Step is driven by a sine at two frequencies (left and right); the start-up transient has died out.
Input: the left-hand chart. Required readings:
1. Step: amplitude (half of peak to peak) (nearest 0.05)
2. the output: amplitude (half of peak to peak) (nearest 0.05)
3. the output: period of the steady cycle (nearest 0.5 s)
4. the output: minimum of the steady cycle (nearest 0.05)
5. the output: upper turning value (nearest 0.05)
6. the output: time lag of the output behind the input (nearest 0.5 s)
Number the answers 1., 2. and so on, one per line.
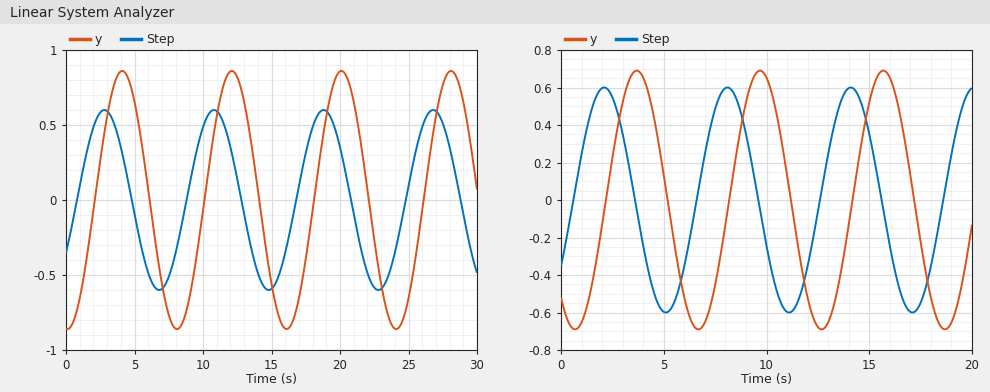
1. 0.60
2. 0.85
3. 8.0 s
4. -0.85
5. 0.85
6. 1.5 s
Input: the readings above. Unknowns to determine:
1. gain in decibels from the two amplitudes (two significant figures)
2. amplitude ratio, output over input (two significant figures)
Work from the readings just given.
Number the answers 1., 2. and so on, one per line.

1. 3.0 dB
2. 1.4
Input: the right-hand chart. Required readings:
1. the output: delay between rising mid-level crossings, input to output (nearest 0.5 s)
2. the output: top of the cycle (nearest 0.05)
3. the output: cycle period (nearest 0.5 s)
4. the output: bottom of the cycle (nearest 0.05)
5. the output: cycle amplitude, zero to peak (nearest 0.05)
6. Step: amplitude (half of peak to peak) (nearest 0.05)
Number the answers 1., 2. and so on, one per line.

1. 1.5 s
2. 0.70
3. 6.0 s
4. -0.70
5. 0.70
6. 0.60
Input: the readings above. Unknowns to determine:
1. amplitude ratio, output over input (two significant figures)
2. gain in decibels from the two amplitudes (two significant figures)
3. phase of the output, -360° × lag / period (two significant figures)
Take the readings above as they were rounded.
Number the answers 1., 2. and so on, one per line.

1. 1.2
2. 1.3 dB
3. -90°
